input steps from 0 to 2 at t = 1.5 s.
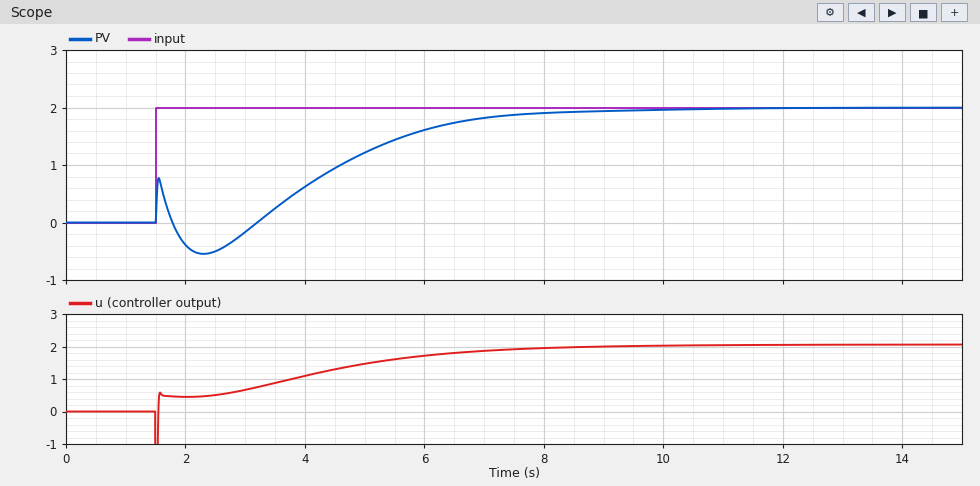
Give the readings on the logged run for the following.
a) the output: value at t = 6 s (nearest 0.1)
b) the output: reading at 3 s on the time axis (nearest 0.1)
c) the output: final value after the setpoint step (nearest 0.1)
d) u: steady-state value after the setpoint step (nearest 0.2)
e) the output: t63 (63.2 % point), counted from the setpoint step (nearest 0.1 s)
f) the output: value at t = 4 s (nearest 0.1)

1.6
-0.2
2.0
2.0
3.6 s
0.6
